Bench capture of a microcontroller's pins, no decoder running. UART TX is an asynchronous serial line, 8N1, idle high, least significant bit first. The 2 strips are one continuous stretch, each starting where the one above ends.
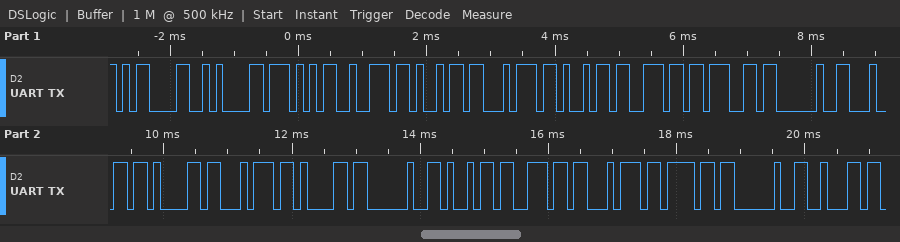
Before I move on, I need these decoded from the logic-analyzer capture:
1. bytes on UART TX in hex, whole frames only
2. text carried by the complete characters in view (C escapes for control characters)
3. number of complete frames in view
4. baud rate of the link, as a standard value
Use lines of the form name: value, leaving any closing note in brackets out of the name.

bytes on UART TX in hex, whole frames only: 0D 0A 57 72 69 74 69 6E 67 20 64 61 74 61 20 69 6E 74 6F 20 62
text carried by the complete characters in view: "\r\nWriting data into b"
number of complete frames in view: 21
baud rate of the link, as a standard value: 9600 baud
